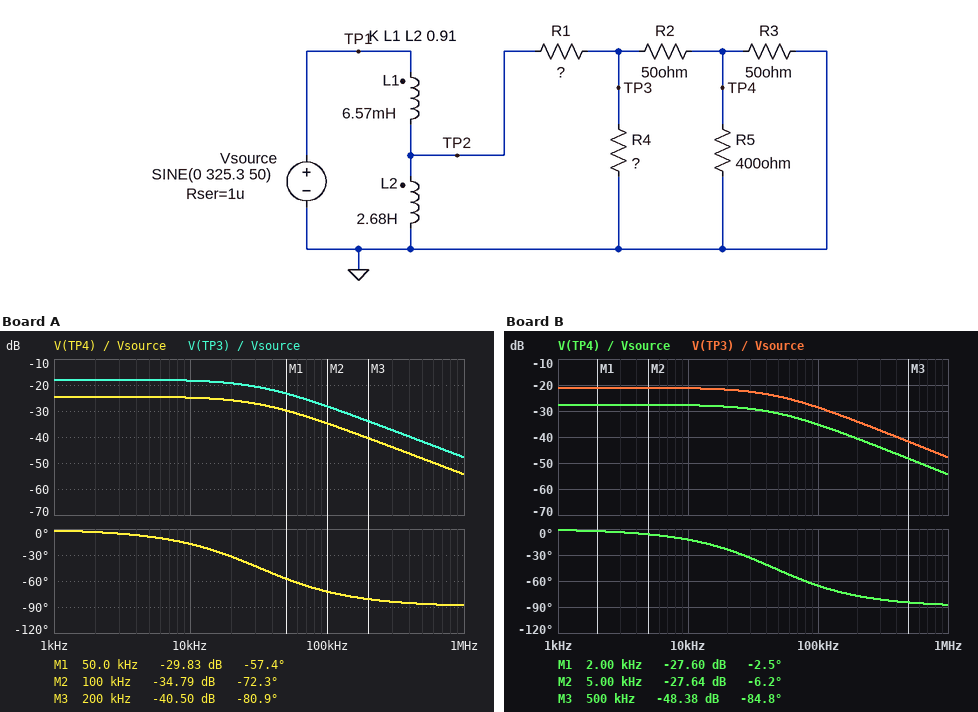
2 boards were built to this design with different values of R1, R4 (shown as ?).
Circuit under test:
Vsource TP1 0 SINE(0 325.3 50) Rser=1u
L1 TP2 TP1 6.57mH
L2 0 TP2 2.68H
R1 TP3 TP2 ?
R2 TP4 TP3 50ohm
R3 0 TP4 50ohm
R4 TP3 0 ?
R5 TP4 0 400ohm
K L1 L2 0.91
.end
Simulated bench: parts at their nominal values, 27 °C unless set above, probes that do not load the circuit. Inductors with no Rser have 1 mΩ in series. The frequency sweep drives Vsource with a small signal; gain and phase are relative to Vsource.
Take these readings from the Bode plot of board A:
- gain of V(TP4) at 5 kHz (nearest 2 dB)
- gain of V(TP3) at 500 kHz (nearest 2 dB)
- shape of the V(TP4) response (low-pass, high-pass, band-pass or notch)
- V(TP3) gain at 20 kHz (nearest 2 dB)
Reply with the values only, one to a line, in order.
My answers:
-24 dB
-42 dB
low-pass
-20 dB
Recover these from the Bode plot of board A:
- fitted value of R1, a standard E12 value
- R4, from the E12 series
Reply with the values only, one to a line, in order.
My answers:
180 Ω
39 Ω
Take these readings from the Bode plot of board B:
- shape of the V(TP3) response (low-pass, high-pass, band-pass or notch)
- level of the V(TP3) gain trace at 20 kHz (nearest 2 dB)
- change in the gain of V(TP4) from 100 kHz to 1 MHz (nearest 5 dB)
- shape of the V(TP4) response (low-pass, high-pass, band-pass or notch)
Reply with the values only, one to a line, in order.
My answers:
low-pass
-22 dB
-20 dB
low-pass
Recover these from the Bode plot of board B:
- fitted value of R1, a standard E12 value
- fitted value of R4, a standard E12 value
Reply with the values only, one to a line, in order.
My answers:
270 Ω
39 Ω
